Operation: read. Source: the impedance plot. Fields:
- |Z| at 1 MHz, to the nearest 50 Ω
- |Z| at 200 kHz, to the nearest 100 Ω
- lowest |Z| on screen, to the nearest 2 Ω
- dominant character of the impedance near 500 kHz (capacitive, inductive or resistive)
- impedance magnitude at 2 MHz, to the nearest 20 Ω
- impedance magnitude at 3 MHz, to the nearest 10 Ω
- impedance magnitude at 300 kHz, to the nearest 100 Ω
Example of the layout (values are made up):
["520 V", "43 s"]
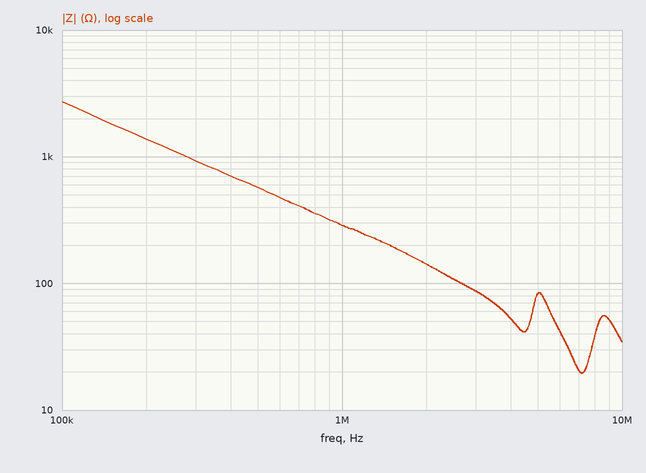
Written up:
["300 Ω", "1.4 kΩ", "20 Ω", "capacitive", "140 Ω", "90 Ω", "900 Ω"]
